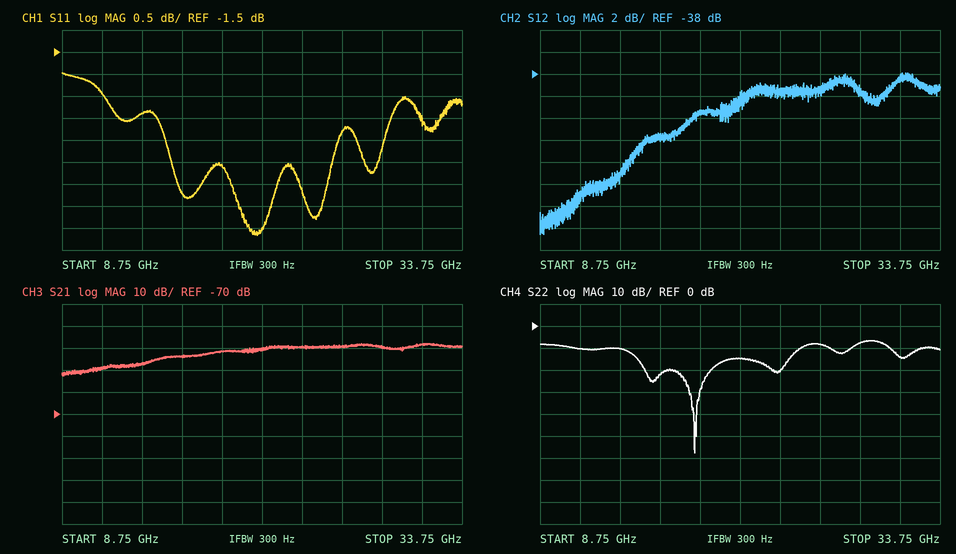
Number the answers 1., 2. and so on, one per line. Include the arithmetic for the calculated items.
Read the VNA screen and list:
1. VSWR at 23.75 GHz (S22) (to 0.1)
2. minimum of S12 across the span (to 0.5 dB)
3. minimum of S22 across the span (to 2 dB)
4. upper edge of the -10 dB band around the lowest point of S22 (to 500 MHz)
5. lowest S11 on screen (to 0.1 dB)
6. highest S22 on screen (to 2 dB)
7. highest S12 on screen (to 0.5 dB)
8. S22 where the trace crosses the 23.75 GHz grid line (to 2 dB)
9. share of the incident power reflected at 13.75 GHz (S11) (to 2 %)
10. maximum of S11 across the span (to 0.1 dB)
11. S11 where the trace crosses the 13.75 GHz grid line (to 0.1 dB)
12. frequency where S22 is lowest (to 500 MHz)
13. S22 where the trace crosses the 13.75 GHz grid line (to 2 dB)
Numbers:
1. |Γ| = 10^(-20/20) = 0.1000; VSWR = (1 + 0.1000)/(1 − 0.1000) ≈ 1.2
2. -52.5 dB
3. -58 dB
4. 25.0 GHz
5. -5.7 dB
6. -6 dB
7. -38.0 dB
8. -20 dB
9. 10^(-2.9/10) ≈ 51.3 %, so 52 % to the nearest 2 %
10. -2.0 dB
11. -2.9 dB
12. 18.5 GHz
13. -10 dB
